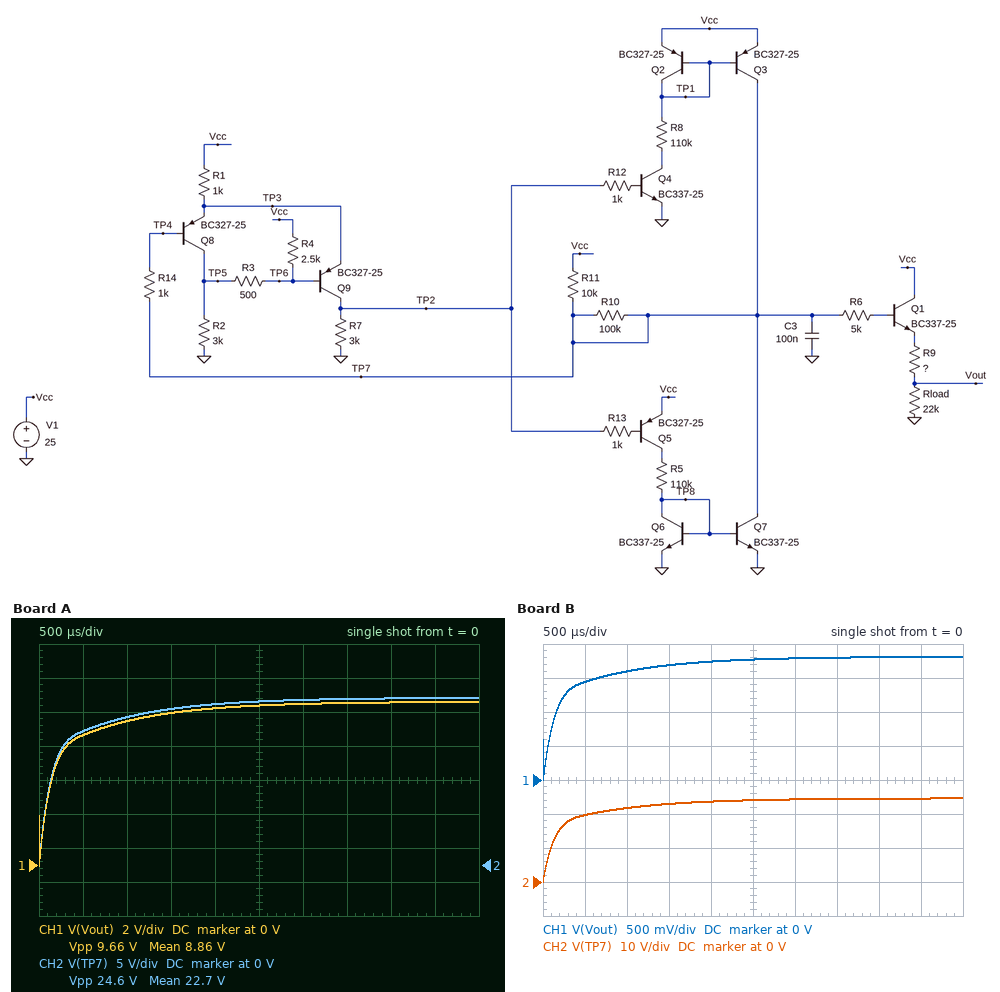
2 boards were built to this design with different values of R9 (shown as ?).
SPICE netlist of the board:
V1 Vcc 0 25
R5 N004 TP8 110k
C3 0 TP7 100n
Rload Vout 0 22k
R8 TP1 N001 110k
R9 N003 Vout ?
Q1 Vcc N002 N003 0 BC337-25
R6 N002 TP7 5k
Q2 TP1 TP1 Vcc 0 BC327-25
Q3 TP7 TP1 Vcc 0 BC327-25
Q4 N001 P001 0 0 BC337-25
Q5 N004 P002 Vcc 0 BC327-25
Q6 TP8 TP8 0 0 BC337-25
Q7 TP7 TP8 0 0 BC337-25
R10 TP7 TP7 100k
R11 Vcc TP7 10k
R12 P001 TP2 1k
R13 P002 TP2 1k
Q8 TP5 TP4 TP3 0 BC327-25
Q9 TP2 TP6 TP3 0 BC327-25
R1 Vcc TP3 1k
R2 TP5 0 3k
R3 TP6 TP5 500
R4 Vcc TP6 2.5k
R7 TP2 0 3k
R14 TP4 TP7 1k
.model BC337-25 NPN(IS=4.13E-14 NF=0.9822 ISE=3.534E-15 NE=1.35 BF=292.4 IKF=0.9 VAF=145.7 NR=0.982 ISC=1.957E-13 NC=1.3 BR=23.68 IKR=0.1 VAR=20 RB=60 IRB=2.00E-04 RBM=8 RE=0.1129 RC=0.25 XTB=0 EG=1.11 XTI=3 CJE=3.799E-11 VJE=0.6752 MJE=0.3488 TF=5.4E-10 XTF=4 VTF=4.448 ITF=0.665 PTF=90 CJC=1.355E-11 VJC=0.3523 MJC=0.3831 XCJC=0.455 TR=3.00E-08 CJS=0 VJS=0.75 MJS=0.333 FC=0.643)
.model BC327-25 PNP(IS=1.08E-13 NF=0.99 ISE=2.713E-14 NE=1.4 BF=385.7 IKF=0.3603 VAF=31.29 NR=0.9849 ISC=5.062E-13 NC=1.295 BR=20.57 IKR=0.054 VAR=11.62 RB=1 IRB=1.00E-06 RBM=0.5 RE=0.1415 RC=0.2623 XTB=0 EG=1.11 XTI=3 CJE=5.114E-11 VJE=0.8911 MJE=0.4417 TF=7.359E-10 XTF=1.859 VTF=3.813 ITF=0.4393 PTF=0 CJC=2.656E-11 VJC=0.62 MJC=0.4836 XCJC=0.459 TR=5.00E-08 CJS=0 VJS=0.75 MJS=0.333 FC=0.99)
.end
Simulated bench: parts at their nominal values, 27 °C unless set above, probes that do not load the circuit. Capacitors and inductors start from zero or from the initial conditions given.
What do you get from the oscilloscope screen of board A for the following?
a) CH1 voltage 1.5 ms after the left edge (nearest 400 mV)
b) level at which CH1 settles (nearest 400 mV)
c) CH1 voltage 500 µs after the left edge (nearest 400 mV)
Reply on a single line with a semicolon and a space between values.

8.8 V; 9.6 V; 7.6 V
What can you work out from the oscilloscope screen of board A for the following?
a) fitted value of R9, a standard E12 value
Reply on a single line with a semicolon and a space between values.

33 kΩ
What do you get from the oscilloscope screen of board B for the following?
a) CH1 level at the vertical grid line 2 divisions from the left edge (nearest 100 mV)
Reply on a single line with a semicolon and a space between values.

1.6 V
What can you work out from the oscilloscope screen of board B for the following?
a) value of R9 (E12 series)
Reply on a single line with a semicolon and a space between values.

270 kΩ
